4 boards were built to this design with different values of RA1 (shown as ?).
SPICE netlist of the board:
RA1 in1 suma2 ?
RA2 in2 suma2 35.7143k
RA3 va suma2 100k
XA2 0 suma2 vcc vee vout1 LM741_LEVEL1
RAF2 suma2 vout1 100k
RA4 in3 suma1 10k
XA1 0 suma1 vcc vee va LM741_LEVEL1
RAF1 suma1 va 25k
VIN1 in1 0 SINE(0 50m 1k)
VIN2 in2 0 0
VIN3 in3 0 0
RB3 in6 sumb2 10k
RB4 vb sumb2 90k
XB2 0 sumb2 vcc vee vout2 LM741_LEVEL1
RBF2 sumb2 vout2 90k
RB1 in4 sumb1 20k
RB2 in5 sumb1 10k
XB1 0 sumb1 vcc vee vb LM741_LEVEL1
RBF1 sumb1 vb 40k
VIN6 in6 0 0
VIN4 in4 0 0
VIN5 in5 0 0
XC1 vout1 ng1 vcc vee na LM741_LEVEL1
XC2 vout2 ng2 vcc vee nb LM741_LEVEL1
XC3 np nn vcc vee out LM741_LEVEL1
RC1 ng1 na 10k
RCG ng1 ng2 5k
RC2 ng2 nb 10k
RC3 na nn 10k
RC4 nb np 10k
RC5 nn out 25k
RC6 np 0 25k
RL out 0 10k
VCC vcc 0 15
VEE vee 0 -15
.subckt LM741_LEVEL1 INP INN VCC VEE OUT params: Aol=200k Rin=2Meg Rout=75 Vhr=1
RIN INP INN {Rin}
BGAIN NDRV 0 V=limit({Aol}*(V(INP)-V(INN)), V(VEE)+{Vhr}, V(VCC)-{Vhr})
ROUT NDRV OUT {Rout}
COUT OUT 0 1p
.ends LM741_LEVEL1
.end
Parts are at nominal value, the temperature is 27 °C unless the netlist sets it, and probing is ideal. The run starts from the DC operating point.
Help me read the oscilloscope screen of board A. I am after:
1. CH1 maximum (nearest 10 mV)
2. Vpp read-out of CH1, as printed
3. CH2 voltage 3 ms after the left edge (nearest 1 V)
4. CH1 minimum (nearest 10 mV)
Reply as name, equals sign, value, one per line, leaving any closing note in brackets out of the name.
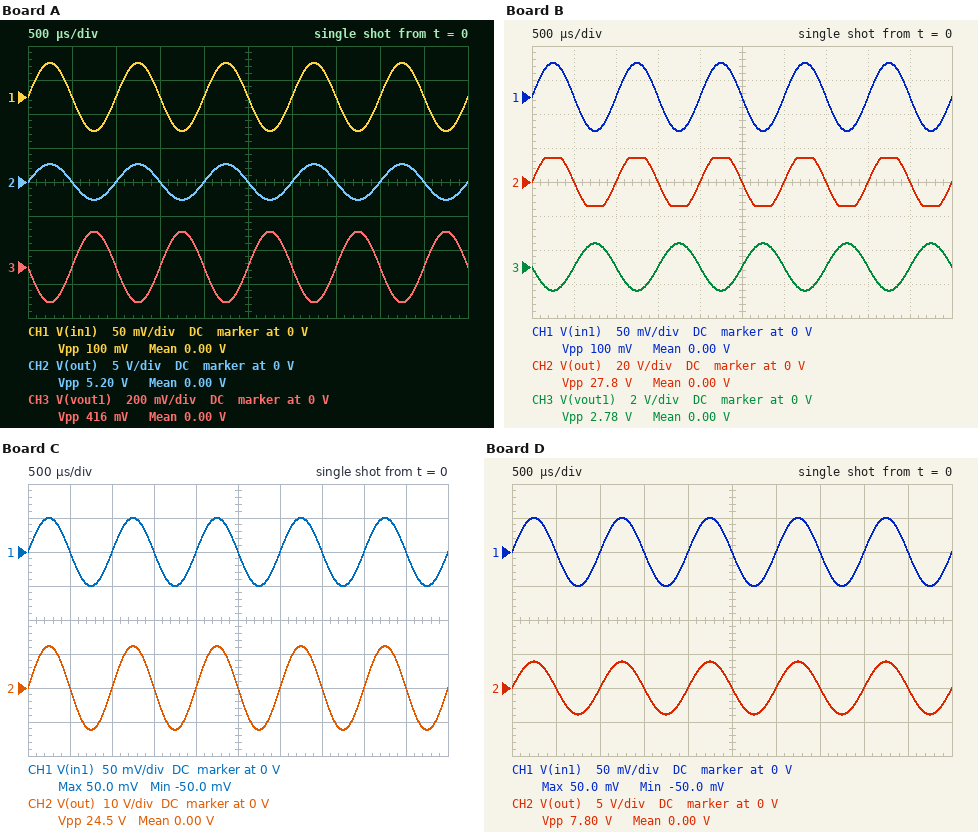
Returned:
CH1 maximum = 50 mV
Vpp read-out of CH1, as printed = 100 mV
CH2 voltage 3 ms after the left edge = 0 V
CH1 minimum = -50 mV
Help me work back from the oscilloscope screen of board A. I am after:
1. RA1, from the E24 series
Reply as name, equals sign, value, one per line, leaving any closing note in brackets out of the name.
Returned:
RA1, from the E24 series = 24 kΩ
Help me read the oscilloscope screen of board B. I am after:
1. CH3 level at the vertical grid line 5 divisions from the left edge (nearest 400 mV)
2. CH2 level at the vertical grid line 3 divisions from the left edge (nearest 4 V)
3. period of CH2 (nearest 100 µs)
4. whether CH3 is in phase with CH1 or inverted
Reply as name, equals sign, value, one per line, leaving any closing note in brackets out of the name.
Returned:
CH3 level at the vertical grid line 5 divisions from the left edge = 0 V
CH2 level at the vertical grid line 3 divisions from the left edge = 0 V
period of CH2 = 1.0 ms
whether CH3 is in phase with CH1 or inverted = inverted
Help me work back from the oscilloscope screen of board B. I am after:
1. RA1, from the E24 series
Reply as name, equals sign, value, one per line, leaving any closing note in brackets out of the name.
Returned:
RA1, from the E24 series = 3.6 kΩ
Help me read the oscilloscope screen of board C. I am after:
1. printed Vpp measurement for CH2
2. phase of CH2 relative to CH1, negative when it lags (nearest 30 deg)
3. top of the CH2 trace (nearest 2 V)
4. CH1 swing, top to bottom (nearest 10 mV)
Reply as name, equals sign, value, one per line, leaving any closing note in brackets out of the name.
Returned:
printed Vpp measurement for CH2 = 24.5 V
phase of CH2 relative to CH1, negative when it lags = 0 deg
top of the CH2 trace = 12 V
CH1 swing, top to bottom = 100 mV
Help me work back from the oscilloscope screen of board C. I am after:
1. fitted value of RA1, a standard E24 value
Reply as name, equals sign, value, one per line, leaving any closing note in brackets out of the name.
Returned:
fitted value of RA1, a standard E24 value = 5.1 kΩ
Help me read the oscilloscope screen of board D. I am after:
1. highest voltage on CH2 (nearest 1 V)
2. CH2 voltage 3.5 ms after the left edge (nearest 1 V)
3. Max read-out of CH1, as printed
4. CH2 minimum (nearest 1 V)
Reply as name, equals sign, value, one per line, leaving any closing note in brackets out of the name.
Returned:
highest voltage on CH2 = 4 V
CH2 voltage 3.5 ms after the left edge = 0 V
Max read-out of CH1, as printed = 50.0 mV
CH2 minimum = -4 V
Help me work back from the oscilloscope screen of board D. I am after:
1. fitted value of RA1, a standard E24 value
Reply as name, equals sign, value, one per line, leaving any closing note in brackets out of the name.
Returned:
fitted value of RA1, a standard E24 value = 16 kΩ
